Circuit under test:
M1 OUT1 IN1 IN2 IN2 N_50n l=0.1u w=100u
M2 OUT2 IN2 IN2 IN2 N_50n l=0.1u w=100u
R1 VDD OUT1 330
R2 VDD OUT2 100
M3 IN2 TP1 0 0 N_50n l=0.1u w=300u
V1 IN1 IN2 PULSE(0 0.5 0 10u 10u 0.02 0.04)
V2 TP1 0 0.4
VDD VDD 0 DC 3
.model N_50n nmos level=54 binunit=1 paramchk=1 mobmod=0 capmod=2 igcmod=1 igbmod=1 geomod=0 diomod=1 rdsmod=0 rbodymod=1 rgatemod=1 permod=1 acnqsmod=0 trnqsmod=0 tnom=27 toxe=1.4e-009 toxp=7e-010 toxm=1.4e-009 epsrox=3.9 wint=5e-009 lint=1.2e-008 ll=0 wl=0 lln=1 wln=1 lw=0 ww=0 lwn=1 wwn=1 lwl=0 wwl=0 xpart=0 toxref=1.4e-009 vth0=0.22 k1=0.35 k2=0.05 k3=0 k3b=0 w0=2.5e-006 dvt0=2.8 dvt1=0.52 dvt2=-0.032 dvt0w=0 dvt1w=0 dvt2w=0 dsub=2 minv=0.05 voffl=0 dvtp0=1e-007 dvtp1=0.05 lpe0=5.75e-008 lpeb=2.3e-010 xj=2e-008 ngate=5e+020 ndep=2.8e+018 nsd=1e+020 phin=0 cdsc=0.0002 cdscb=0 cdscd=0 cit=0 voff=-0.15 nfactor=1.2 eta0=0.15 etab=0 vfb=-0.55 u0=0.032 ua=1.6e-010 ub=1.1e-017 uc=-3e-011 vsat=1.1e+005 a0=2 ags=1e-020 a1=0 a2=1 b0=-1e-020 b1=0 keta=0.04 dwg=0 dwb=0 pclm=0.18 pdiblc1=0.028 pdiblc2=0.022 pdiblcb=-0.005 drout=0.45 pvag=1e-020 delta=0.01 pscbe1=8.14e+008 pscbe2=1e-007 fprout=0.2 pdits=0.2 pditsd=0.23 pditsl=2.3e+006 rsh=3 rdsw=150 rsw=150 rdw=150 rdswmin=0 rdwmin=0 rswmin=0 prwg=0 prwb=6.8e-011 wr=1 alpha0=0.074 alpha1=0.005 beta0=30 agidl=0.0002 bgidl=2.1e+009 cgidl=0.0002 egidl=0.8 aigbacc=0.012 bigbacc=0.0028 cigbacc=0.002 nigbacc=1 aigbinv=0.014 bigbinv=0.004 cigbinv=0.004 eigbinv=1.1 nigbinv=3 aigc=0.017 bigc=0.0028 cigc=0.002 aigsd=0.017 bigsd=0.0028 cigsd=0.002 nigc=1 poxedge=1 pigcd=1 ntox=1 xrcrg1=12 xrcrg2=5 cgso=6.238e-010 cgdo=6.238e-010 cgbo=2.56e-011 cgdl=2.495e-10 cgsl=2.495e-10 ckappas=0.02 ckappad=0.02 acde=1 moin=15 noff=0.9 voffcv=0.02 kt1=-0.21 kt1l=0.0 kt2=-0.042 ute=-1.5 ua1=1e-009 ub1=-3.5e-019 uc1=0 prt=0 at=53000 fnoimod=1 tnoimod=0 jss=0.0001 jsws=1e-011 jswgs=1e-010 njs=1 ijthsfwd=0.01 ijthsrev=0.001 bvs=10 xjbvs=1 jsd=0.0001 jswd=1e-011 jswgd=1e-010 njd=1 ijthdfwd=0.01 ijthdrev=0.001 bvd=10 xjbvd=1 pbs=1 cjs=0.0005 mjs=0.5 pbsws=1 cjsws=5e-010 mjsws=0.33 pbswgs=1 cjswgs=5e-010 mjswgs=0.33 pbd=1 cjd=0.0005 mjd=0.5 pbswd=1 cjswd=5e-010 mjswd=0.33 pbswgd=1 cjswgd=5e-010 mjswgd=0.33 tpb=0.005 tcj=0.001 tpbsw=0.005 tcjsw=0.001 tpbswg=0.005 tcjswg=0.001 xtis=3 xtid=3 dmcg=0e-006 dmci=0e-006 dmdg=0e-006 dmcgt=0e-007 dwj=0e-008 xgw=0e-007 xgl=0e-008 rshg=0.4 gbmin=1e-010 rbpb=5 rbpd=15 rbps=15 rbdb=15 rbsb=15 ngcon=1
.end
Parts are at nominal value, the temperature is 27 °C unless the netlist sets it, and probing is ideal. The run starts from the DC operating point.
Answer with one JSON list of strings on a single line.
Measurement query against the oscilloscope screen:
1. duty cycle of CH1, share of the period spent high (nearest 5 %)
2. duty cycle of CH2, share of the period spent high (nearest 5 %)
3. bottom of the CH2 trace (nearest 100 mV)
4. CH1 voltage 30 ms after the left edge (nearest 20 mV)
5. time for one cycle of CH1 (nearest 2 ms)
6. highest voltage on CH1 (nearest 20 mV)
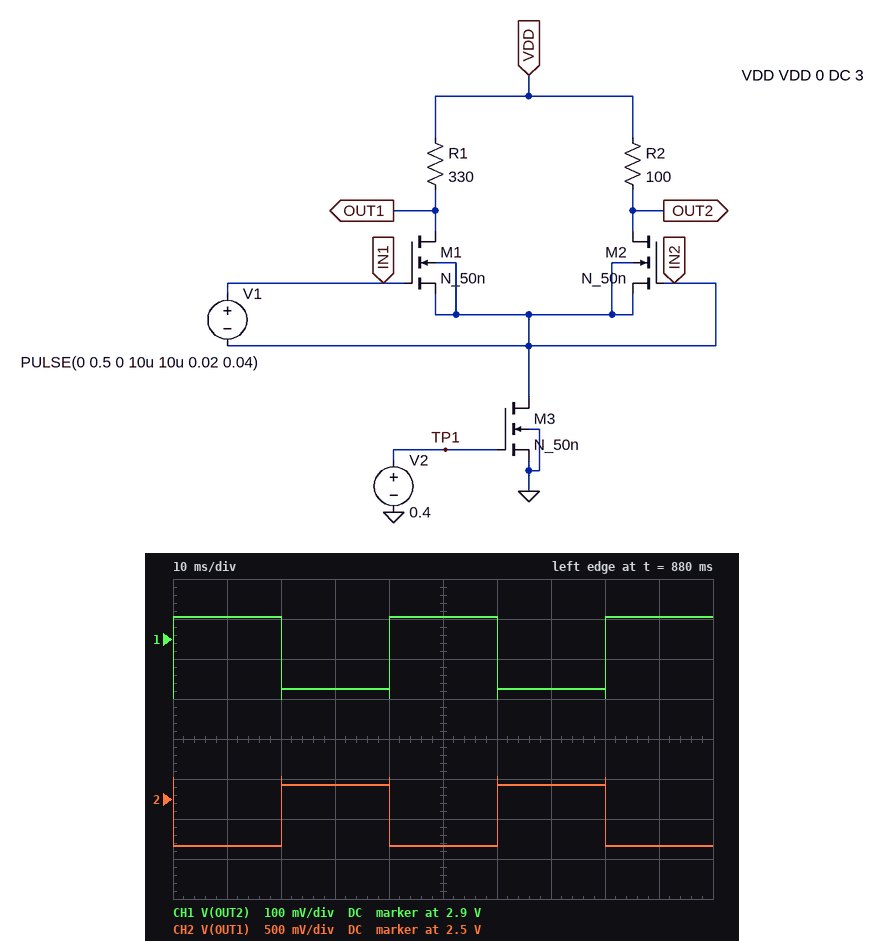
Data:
["50 %", "50 %", "1.9 V", "2.78 V", "40 ms", "2.96 V"]
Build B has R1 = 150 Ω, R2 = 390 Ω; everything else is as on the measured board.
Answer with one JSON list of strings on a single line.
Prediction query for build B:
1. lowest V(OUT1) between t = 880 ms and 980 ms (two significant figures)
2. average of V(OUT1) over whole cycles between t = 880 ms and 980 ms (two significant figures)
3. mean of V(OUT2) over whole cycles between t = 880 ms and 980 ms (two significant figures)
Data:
["2.4 V", "2.6 V", "2.8 V"]
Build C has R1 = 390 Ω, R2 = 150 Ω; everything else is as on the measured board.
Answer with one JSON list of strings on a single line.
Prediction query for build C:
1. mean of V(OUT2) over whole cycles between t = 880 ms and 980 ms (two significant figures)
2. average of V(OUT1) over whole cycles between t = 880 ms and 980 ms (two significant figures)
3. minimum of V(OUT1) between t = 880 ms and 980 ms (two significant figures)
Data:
["2.8 V", "2.2 V", "1.8 V"]
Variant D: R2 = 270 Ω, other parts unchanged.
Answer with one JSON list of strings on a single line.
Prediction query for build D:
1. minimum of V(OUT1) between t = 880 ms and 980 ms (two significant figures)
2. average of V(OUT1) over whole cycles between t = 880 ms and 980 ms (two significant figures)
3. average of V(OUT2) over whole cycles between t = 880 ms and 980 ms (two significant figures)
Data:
["1.9 V", "2.2 V", "2.7 V"]
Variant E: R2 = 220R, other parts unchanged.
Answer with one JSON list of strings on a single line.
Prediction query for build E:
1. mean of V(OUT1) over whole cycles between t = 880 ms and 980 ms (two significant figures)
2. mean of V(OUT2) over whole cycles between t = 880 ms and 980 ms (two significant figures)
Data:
["2.2 V", "2.8 V"]
